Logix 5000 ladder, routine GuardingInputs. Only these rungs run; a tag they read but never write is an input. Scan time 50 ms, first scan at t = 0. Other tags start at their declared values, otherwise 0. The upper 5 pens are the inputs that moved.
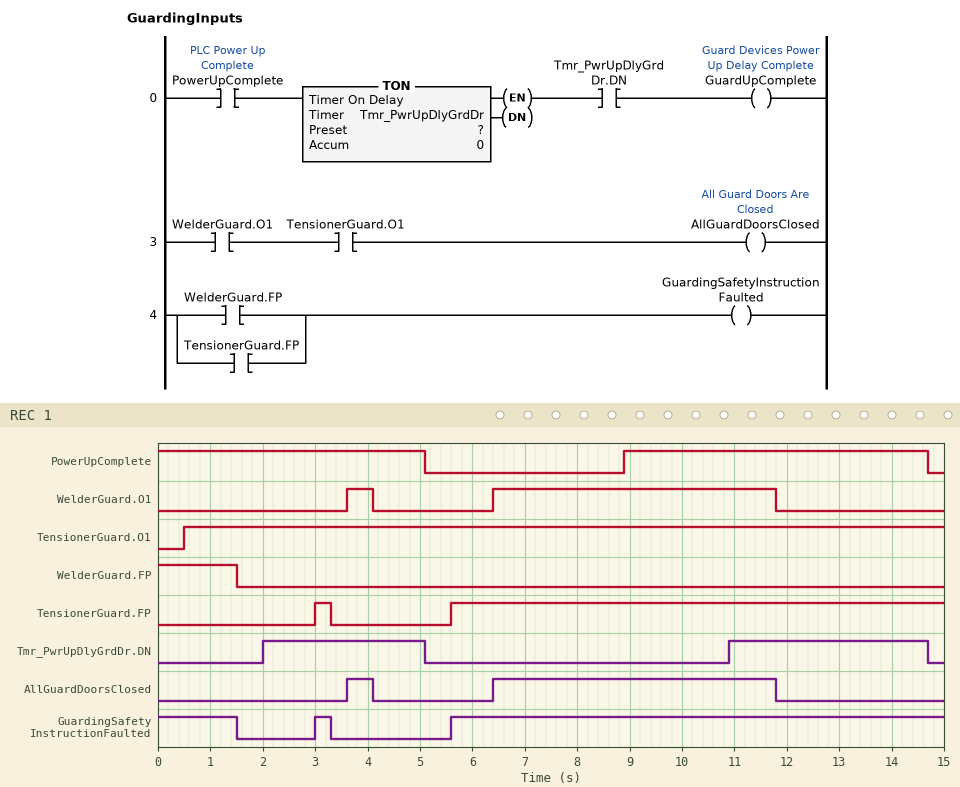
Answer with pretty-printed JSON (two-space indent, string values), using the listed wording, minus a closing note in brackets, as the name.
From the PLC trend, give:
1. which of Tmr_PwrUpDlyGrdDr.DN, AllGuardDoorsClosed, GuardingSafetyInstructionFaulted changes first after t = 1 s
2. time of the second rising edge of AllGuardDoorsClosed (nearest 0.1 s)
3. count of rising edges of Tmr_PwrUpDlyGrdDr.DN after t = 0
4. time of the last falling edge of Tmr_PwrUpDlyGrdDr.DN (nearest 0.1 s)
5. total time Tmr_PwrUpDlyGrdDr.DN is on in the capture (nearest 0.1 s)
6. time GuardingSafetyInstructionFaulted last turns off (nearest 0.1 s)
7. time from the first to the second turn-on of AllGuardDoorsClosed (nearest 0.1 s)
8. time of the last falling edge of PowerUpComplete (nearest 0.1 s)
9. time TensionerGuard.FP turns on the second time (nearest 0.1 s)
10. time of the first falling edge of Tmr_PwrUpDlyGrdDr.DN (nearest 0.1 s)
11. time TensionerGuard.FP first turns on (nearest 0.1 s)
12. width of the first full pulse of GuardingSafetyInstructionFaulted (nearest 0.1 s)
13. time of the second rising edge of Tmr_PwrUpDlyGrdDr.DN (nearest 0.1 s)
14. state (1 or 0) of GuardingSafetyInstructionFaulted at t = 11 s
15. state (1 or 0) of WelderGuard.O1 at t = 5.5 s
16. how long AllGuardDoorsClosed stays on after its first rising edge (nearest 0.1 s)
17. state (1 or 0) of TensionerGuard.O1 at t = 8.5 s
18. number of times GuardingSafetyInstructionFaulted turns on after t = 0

{
  "which of Tmr_PwrUpDlyGrdDr.DN, AllGuardDoorsClosed, GuardingSafetyInstructionFaulted changes first after t = 1 s": "GuardingSafetyInstructionFaulted",
  "time of the second rising edge of AllGuardDoorsClosed": "6.4 s",
  "count of rising edges of Tmr_PwrUpDlyGrdDr.DN after t = 0": "2",
  "time of the last falling edge of Tmr_PwrUpDlyGrdDr.DN": "14.7 s",
  "total time Tmr_PwrUpDlyGrdDr.DN is on in the capture": "6.9 s",
  "time GuardingSafetyInstructionFaulted last turns off": "3.3 s",
  "time from the first to the second turn-on of AllGuardDoorsClosed": "2.8 s",
  "time of the last falling edge of PowerUpComplete": "14.7 s",
  "time TensionerGuard.FP turns on the second time": "5.6 s",
  "time of the first falling edge of Tmr_PwrUpDlyGrdDr.DN": "5.1 s",
  "time TensionerGuard.FP first turns on": "3.0 s",
  "width of the first full pulse of GuardingSafetyInstructionFaulted": "0.3 s",
  "time of the second rising edge of Tmr_PwrUpDlyGrdDr.DN": "10.9 s",
  "state (1 or 0) of GuardingSafetyInstructionFaulted at t = 11 s": "1",
  "state (1 or 0) of WelderGuard.O1 at t = 5.5 s": "0",
  "how long AllGuardDoorsClosed stays on after its first rising edge": "0.5 s",
  "state (1 or 0) of TensionerGuard.O1 at t = 8.5 s": "1",
  "number of times GuardingSafetyInstructionFaulted turns on after t = 0": "2"
}
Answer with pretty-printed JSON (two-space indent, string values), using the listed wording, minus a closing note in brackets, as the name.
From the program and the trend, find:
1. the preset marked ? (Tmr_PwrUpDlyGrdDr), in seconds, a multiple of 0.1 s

{
  "the preset marked ? (Tmr_PwrUpDlyGrdDr), in seconds, a multiple of 0.1 s": "2.0 s"
}
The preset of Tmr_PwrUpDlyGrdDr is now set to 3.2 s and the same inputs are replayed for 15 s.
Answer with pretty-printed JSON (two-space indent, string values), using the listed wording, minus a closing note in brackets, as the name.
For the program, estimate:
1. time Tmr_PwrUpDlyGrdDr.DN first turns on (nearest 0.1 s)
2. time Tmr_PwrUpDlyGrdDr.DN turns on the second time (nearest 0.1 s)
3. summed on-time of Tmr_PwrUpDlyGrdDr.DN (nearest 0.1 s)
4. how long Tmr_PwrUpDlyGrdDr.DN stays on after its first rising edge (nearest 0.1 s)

{
  "time Tmr_PwrUpDlyGrdDr.DN first turns on": "3.2 s",
  "time Tmr_PwrUpDlyGrdDr.DN turns on the second time": "12.1 s",
  "summed on-time of Tmr_PwrUpDlyGrdDr.DN": "4.5 s",
  "how long Tmr_PwrUpDlyGrdDr.DN stays on after its first rising edge": "1.9 s"
}
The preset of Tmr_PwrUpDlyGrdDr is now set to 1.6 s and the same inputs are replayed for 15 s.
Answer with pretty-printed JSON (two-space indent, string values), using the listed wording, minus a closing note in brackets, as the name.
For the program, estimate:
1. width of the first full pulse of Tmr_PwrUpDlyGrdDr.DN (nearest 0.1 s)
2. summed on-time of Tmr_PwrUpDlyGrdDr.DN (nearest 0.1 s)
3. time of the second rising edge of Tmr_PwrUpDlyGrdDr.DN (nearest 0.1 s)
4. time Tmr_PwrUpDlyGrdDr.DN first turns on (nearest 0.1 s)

{
  "width of the first full pulse of Tmr_PwrUpDlyGrdDr.DN": "3.5 s",
  "summed on-time of Tmr_PwrUpDlyGrdDr.DN": "7.7 s",
  "time of the second rising edge of Tmr_PwrUpDlyGrdDr.DN": "10.5 s",
  "time Tmr_PwrUpDlyGrdDr.DN first turns on": "1.6 s"
}
